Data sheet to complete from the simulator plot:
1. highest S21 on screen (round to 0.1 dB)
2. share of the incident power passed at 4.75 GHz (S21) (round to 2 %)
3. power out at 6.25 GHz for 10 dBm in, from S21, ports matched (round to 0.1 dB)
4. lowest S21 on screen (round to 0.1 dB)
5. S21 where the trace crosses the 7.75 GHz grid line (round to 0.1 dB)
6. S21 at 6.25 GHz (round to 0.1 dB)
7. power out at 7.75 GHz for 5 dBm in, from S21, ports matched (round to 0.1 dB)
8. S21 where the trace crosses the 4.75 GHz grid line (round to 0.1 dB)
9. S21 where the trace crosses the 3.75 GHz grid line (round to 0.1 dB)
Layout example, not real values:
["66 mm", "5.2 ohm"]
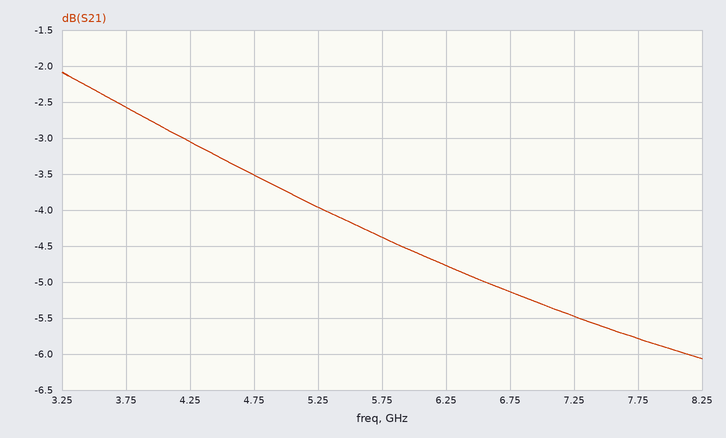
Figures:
["-2.1 dB", "44 %", "5.2 dBm", "-6.1 dB", "-5.8 dB", "-4.8 dB", "-0.8 dBm", "-3.5 dB", "-2.6 dB"]
